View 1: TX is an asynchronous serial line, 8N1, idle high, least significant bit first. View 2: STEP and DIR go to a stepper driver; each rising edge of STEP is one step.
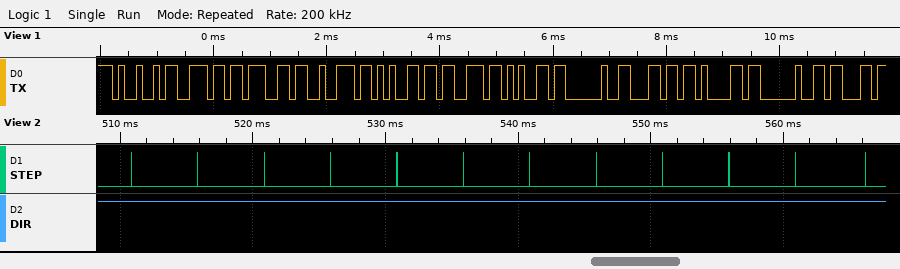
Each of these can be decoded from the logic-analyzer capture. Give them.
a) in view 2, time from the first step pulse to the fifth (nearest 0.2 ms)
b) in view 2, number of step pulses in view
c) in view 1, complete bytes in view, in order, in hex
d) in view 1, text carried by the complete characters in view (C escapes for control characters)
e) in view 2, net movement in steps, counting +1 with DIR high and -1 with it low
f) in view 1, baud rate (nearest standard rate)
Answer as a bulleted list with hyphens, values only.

- 20.0 ms
- 12
- 49 6E 67 72 65 73 65 20 6C 61 20 63
- "Ingrese la c"
- +12
- 9600 baud
